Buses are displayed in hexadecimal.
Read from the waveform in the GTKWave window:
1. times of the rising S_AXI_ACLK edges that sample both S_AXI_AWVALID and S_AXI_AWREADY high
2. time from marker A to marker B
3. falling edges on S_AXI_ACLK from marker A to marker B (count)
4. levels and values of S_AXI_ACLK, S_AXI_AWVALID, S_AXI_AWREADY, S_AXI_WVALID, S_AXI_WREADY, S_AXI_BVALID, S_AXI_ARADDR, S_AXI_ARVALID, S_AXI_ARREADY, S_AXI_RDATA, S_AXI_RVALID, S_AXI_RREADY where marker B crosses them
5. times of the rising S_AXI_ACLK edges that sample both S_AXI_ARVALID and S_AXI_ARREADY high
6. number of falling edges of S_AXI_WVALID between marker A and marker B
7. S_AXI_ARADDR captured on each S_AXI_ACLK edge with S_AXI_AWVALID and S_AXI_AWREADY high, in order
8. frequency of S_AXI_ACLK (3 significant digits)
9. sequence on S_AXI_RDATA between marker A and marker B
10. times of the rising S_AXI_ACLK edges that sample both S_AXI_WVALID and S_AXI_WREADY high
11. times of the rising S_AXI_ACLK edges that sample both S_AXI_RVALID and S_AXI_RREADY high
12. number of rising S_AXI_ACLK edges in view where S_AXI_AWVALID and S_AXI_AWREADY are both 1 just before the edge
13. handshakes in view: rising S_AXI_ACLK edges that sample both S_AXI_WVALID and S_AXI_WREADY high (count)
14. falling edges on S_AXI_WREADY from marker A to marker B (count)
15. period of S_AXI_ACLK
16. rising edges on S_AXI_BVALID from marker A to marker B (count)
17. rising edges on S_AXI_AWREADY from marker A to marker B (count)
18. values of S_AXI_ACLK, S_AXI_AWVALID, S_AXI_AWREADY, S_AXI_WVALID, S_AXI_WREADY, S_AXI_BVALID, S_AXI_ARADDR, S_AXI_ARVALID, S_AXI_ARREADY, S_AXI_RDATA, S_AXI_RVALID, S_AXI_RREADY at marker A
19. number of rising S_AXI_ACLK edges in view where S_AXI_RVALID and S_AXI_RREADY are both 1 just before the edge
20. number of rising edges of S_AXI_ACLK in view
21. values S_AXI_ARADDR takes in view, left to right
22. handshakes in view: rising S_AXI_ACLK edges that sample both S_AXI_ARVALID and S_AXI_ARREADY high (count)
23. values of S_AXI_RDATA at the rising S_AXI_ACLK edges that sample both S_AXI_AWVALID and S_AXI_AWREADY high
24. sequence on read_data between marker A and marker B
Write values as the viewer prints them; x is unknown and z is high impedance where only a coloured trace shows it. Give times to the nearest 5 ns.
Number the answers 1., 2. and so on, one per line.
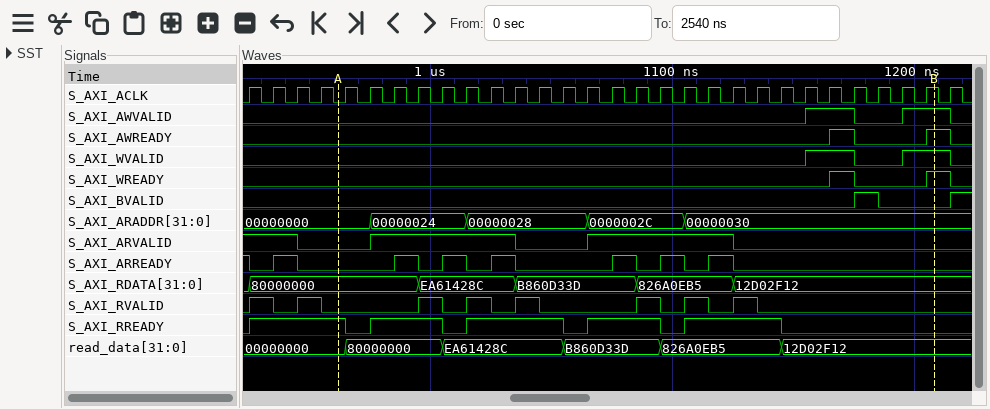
1. 1175 ns, 1215 ns
2. 245 ns
3. 24
4. S_AXI_ACLK=1, S_AXI_AWVALID=1, S_AXI_AWREADY=1, S_AXI_WVALID=1, S_AXI_WREADY=1, S_AXI_BVALID=0, S_AXI_ARADDR=00000030, S_AXI_ARVALID=0, S_AXI_ARREADY=0, S_AXI_RDATA=12D02F12, S_AXI_RVALID=0, S_AXI_RREADY=0
5. 925 ns, 945 ns, 995 ns, 1015 ns, 1035 ns, 1085 ns, 1105 ns, 1125 ns
6. 1
7. 00000030, 00000030
8. 100 MHz
9. 80000000, EA61428C, B860D33D, 826A0EB5, 12D02F12
10. 1175 ns, 1215 ns
11. 935 ns, 955 ns, 1005 ns, 1025 ns, 1045 ns, 1095 ns, 1115 ns, 1135 ns
12. 2
13. 2
14. 1
15. 10 ns
16. 1
17. 2
18. S_AXI_ACLK=0, S_AXI_AWVALID=0, S_AXI_AWREADY=0, S_AXI_WVALID=0, S_AXI_WREADY=0, S_AXI_BVALID=0, S_AXI_ARADDR=00000000, S_AXI_ARVALID=0, S_AXI_ARREADY=0, S_AXI_RDATA=80000000, S_AXI_RVALID=0, S_AXI_RREADY=1
19. 8
20. 30
21. 00000000, 00000024, 00000028, 0000002C, 00000030
22. 8
23. 12D02F12, 12D02F12
24. 00000000, 80000000, EA61428C, B860D33D, 826A0EB5, 12D02F12
